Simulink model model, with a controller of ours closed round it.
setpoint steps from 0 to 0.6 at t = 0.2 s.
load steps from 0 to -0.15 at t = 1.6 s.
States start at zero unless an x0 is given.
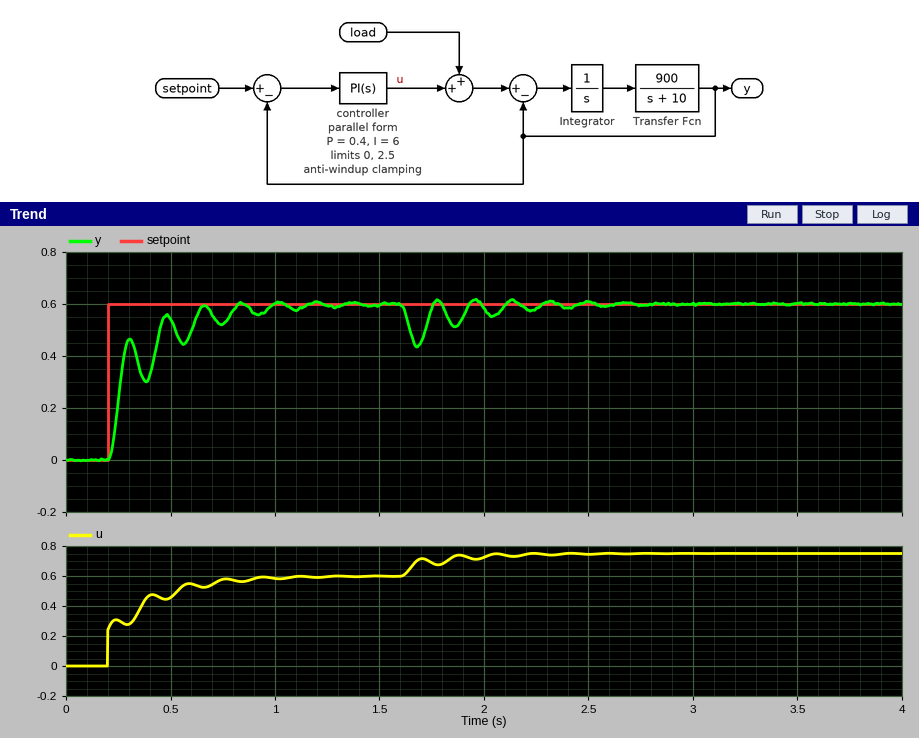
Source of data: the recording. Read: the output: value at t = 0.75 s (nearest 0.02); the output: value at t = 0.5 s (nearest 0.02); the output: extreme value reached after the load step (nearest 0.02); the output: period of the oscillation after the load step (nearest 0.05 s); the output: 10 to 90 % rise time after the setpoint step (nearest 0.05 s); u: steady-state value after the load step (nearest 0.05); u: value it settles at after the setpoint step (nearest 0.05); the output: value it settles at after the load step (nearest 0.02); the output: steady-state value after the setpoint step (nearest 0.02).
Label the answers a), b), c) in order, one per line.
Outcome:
a) 0.52
b) 0.54
c) 0.44
d) 0.20 s
e) 0.25 s
f) 0.75
g) 0.60
h) 0.60
i) 0.60
